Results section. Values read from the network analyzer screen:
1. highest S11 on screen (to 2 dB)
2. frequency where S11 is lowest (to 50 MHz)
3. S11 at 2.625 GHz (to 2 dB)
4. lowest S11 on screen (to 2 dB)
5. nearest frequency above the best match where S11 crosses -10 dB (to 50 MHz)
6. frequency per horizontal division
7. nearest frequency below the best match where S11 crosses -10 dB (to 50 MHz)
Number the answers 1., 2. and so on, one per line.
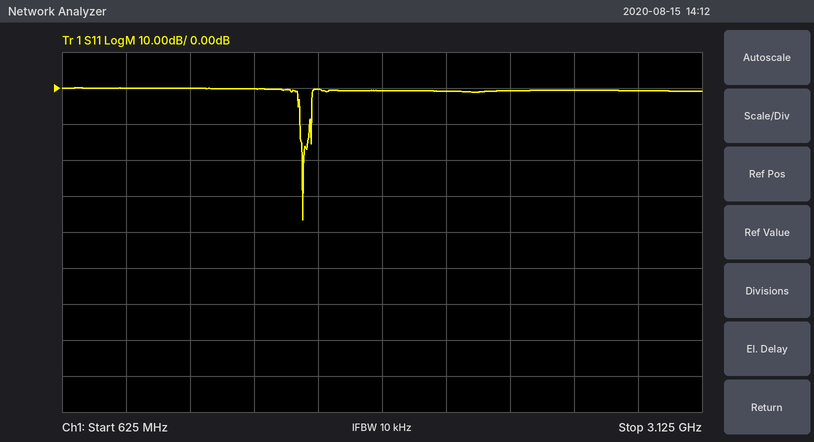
1. 0 dB
2. 1.55 GHz
3. 0 dB
4. -36 dB
5. 1.60 GHz
6. 250 MHz
7. 1.55 GHz
